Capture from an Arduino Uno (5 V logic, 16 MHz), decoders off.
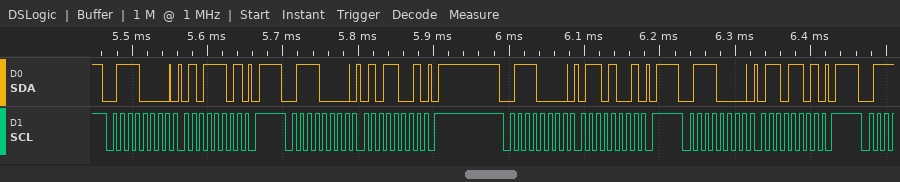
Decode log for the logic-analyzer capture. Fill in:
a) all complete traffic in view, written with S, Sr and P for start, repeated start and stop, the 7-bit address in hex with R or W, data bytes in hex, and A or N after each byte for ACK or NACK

S 38W A 5D A P S 38W A 59 A P S 38W A 69 A P S 38W A 6D A P
